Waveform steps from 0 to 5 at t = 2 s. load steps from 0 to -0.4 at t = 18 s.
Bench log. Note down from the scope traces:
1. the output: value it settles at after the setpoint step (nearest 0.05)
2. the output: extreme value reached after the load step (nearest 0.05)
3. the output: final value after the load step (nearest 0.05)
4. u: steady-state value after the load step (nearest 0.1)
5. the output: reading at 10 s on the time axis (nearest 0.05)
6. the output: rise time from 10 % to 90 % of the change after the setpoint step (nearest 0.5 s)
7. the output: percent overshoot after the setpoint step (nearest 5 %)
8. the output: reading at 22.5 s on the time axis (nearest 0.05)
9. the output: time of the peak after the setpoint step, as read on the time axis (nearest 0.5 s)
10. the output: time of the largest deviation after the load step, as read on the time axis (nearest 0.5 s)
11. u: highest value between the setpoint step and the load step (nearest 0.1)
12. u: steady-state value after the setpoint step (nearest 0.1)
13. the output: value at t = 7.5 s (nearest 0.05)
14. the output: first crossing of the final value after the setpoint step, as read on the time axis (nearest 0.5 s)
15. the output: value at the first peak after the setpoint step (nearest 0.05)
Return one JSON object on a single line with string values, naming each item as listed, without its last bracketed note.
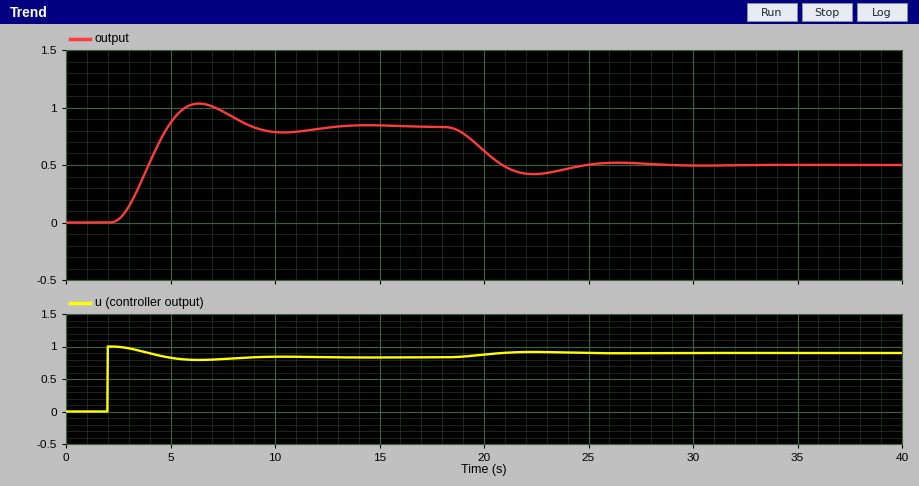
{"the output: value it settles at after the setpoint step": "0.85", "the output: extreme value reached after the load step": "0.40", "the output: final value after the load step": "0.50", "u: steady-state value after the load step": "0.9", "the output: reading at 10 s on the time axis": "0.80", "the output: rise time from 10 % to 90 % of the change after the setpoint step": "2.0 s", "the output: percent overshoot after the setpoint step": "25 %", "the output: reading at 22.5 s on the time axis": "0.40", "the output: time of the peak after the setpoint step, as read on the time axis": "6.5 s", "the output: time of the largest deviation after the load step, as read on the time axis": "22.5 s", "u: highest value between the setpoint step and the load step": "1.0", "u: steady-state value after the setpoint step": "0.8", "the output: value at t = 7.5 s": "0.95", "the output: first crossing of the final value after the setpoint step, as read on the time axis": "5.0 s", "the output: value at the first peak after the setpoint step": "1.05"}
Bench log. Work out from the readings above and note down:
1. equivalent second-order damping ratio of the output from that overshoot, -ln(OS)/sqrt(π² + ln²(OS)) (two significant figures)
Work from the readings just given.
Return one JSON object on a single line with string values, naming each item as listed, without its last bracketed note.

{"equivalent second-order damping ratio of the output from that overshoot, -ln(OS)/sqrt(π² + ln²(OS))": "0.40"}
